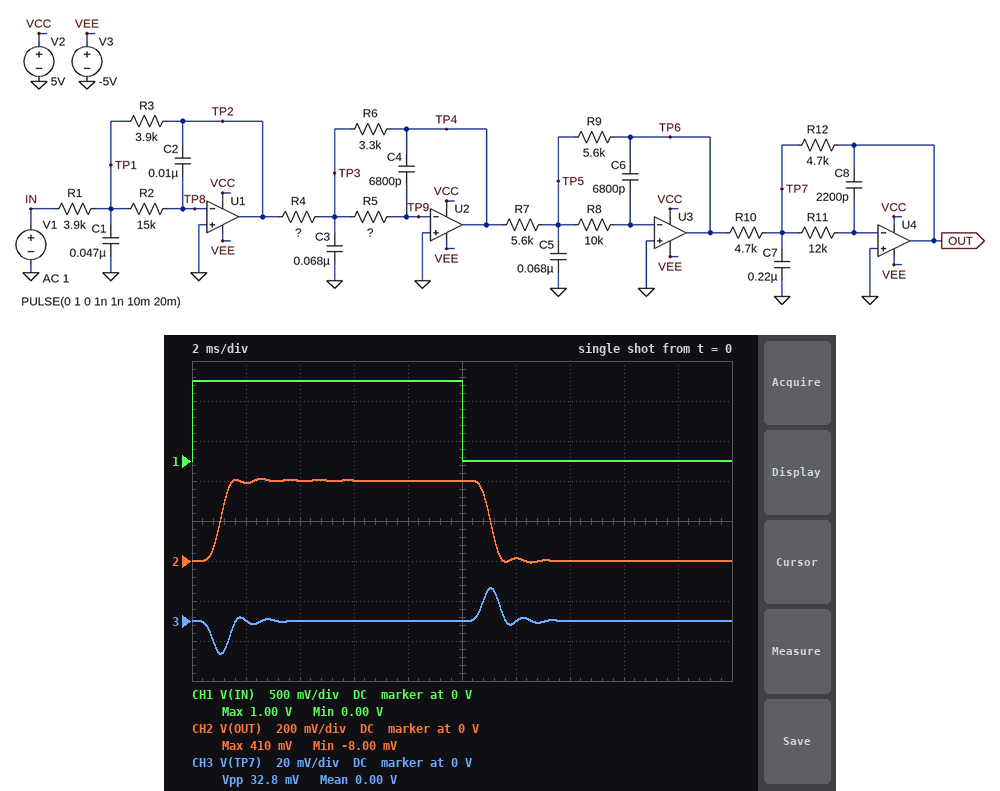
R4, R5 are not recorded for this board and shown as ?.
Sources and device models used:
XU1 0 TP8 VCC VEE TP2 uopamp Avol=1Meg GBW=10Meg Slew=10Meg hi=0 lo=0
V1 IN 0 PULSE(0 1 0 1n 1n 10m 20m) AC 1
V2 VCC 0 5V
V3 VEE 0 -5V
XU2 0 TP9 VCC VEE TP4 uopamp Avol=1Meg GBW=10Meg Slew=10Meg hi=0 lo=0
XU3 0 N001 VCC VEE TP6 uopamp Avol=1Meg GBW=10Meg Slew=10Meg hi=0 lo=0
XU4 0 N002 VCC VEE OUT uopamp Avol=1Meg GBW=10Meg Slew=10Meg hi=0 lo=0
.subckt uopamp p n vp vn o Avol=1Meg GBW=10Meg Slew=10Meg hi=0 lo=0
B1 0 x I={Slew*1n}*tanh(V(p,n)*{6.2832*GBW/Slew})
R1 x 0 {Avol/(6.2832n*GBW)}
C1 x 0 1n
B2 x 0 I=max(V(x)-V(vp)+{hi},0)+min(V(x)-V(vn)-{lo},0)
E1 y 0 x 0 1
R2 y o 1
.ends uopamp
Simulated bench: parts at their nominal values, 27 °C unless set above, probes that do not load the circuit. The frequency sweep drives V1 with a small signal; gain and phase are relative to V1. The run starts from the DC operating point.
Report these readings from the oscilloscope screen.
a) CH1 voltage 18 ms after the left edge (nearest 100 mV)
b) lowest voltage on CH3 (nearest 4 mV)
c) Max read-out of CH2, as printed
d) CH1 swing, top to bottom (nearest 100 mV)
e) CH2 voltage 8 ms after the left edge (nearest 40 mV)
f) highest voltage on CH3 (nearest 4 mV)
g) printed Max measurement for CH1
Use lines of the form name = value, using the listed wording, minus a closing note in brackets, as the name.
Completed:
CH1 voltage 18 ms after the left edge = 0 V
lowest voltage on CH3 = -16 mV
Max read-out of CH2, as printed = 410 mV
CH1 swing, top to bottom = 1.0 V
CH2 voltage 8 ms after the left edge = 400 mV
highest voltage on CH3 = 16 mV
printed Max measurement for CH1 = 1.00 V
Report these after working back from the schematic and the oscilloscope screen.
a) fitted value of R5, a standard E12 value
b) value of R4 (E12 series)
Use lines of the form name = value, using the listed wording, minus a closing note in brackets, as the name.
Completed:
fitted value of R5, a standard E12 value = 47 kΩ
value of R4 = 8.2 kΩ
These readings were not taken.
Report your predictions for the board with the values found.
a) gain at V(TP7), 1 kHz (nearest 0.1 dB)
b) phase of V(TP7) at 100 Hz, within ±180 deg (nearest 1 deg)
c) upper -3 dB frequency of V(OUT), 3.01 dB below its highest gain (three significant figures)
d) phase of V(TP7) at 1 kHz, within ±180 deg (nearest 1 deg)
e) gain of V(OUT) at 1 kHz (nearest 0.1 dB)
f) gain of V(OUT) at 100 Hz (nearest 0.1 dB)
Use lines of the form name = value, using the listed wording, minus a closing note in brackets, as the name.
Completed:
gain at V(TP7), 1 kHz = -33.8 dB
phase of V(TP7) at 100 Hz, within ±180 deg = -128 deg
upper -3 dB frequency of V(OUT), 3.01 dB below its highest gain = 539 Hz
phase of V(TP7) at 1 kHz, within ±180 deg = -136 deg
gain of V(OUT) at 1 kHz = -18.2 dB
gain of V(OUT) at 100 Hz = -8.0 dB
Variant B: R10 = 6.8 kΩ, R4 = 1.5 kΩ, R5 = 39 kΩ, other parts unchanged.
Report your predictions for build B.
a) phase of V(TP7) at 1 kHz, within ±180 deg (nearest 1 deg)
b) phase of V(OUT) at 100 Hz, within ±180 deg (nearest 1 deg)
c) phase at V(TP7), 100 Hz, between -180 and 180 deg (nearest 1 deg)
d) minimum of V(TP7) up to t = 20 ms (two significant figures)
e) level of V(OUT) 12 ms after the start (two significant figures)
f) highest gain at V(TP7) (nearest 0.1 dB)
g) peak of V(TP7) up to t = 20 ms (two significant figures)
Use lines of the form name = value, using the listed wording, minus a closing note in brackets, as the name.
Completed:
phase of V(TP7) at 1 kHz, within ±180 deg = -120 deg
phase of V(OUT) at 100 Hz, within ±180 deg = -50 deg
phase at V(TP7), 100 Hz, between -180 and 180 deg = -140 deg
minimum of V(TP7) up to t = 20 ms = -42 mV
level of V(OUT) 12 ms after the start = 310 mV
highest gain at V(TP7) = -23.0 dB
peak of V(TP7) up to t = 20 ms = 42 mV
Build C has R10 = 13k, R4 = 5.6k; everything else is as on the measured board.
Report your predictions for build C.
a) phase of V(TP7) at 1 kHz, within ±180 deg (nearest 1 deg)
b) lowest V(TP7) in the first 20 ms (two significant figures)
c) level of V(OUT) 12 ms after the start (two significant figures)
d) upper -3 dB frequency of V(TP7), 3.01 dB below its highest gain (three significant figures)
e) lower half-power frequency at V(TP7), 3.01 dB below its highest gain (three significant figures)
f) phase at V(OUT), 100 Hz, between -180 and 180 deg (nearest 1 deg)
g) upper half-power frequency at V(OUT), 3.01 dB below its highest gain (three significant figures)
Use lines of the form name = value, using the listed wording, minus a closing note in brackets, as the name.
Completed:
phase of V(TP7) at 1 kHz, within ±180 deg = -137 deg
lowest V(TP7) in the first 20 ms = -8.4 mV
level of V(OUT) 12 ms after the start = 15 mV
upper -3 dB frequency of V(TP7), 3.01 dB below its highest gain = 1.01 kHz
lower half-power frequency at V(TP7), 3.01 dB below its highest gain = 550 Hz
phase at V(OUT), 100 Hz, between -180 and 180 deg = -39 deg
upper half-power frequency at V(OUT), 3.01 dB below its highest gain = 443 Hz
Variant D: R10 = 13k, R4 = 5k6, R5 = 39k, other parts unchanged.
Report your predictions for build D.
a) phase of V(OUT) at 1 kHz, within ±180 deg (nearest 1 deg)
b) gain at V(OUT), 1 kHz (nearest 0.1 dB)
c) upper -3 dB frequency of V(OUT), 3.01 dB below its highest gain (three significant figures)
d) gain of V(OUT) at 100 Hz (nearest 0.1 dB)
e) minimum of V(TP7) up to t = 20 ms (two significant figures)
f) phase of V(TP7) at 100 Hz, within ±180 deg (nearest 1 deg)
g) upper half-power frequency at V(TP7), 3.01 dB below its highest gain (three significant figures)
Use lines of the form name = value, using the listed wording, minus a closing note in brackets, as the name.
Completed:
phase of V(OUT) at 1 kHz, within ±180 deg = -44 deg
gain at V(OUT), 1 kHz = -20.2 dB
upper -3 dB frequency of V(OUT), 3.01 dB below its highest gain = 651 Hz
gain of V(OUT) at 100 Hz = -13.5 dB
minimum of V(TP7) up to t = 20 ms = -9.4 mV
phase of V(TP7) at 100 Hz, within ±180 deg = -126 deg
upper half-power frequency at V(TP7), 3.01 dB below its highest gain = 1.01 kHz
